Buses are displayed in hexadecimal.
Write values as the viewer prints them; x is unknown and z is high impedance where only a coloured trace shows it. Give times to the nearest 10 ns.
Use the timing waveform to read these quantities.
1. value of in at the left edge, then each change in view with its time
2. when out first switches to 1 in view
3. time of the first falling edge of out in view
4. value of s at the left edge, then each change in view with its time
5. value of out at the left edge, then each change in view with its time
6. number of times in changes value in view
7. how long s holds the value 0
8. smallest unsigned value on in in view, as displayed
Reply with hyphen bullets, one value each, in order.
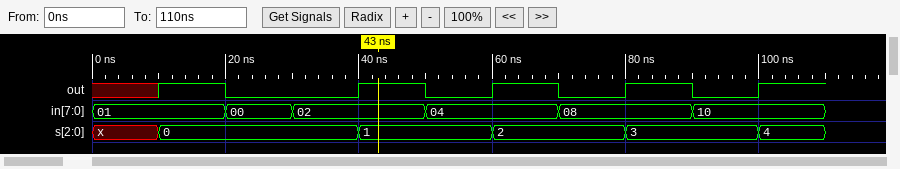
- 01, 00 at 20 ns, 02 at 30 ns, 04 at 50 ns, 08 at 70 ns, 10 at 90 ns
- 10 ns
- 20 ns
- x, 0 at 10 ns, 1 at 40 ns, 2 at 60 ns, 3 at 80 ns, 4 at 100 ns
- x, 1 at 10 ns, 0 at 20 ns, 1 at 40 ns, 0 at 50 ns, 1 at 60 ns, 0 at 70 ns, 1 at 80 ns, 0 at 90 ns, 1 at 100 ns
- 5
- 30 ns
- 00
